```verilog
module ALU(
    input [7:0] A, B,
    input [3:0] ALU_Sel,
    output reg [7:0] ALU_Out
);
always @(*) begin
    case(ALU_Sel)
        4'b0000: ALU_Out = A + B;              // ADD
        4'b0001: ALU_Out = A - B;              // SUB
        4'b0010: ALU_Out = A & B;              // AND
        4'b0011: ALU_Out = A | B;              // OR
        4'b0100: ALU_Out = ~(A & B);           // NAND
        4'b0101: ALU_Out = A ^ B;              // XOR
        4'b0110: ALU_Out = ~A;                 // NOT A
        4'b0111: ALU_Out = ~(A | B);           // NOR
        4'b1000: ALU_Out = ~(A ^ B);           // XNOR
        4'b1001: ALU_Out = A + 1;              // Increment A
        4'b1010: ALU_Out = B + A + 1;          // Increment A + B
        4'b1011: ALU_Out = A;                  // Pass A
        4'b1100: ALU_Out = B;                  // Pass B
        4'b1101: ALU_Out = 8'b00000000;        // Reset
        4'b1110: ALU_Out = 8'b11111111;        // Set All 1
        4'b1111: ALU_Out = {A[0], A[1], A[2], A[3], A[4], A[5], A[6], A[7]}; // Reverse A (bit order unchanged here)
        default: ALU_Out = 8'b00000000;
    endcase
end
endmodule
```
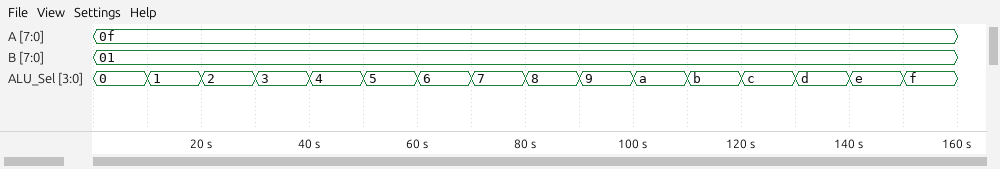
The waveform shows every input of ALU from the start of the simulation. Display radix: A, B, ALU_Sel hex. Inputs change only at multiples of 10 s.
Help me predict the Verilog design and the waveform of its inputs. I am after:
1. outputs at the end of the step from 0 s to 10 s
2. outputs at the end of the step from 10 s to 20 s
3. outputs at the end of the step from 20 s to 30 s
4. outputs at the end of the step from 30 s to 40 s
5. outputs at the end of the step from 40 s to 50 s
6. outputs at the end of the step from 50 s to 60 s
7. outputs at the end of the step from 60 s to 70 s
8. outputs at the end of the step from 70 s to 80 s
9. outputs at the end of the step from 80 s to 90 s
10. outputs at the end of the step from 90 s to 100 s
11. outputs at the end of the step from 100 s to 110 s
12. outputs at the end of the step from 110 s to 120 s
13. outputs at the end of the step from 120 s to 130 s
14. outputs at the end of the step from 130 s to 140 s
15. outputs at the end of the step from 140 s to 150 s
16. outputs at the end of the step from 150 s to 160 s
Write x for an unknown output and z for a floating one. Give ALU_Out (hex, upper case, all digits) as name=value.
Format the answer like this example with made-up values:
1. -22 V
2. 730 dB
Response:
1. ALU_Out=10
2. ALU_Out=0E
3. ALU_Out=01
4. ALU_Out=0F
5. ALU_Out=FE
6. ALU_Out=0E
7. ALU_Out=F0
8. ALU_Out=F0
9. ALU_Out=F1
10. ALU_Out=10
11. ALU_Out=11
12. ALU_Out=0F
13. ALU_Out=01
14. ALU_Out=00
15. ALU_Out=FF
16. ALU_Out=F0
